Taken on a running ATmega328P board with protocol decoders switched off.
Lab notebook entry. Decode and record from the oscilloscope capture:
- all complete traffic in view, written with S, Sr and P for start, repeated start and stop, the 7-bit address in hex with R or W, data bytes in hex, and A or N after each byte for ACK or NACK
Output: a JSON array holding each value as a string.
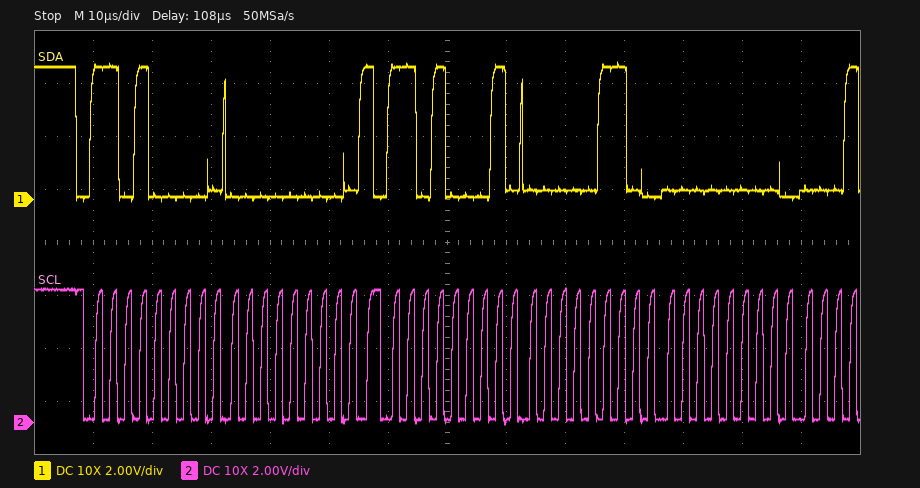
["S 68W A 00 A Sr 68R A 06 A 00 A"]
